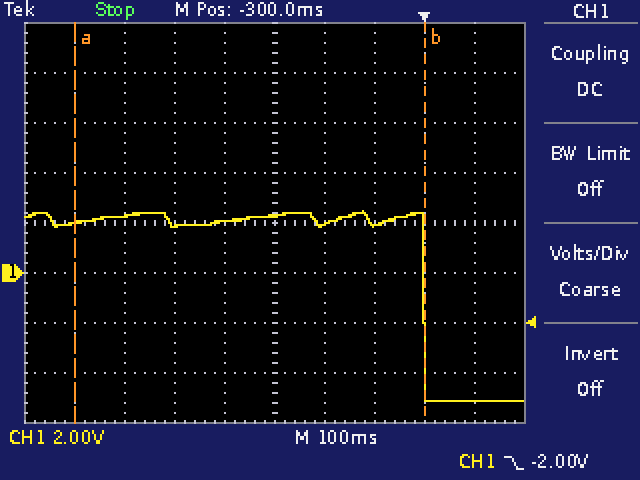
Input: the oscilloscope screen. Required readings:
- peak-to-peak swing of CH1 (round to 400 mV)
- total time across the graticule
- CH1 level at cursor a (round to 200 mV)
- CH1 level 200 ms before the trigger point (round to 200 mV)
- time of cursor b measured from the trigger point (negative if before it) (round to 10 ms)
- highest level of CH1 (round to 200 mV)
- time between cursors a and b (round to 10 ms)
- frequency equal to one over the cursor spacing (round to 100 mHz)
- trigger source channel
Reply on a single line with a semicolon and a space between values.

7.6 V; 1 s; 2.0 V; 2.0 V; 0 ms; 2.4 V; 700 ms; 1.4 Hz; CH1
